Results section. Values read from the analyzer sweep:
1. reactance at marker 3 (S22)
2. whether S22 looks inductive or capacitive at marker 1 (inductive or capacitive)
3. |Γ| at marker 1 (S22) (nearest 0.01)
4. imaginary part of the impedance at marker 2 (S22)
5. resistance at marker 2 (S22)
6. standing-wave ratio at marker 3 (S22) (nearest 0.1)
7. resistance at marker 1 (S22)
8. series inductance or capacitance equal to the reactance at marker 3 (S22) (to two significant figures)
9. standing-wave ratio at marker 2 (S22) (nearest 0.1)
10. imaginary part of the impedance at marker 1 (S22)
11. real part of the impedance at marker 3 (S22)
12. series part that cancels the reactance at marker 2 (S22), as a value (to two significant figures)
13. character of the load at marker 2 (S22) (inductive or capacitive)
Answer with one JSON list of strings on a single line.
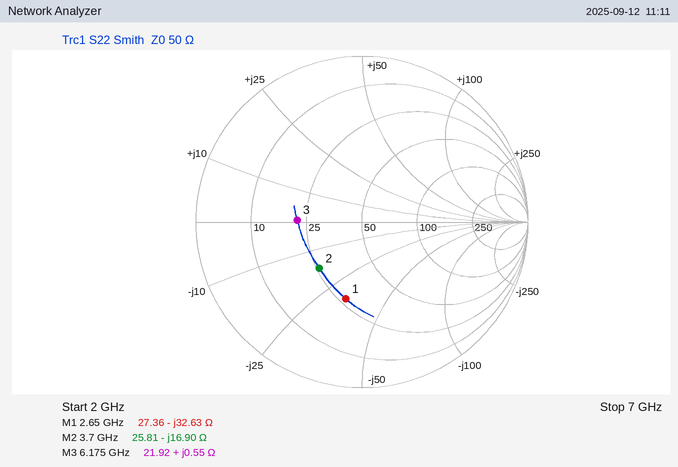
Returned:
["+0.55 Ω", "capacitive", "0.47", "-16.90 Ω", "25.81 Ω", "2.3", "27.36 Ω", "14 pH", "2.2", "-32.63 Ω", "21.92 Ω", "730 pH", "capacitive"]
